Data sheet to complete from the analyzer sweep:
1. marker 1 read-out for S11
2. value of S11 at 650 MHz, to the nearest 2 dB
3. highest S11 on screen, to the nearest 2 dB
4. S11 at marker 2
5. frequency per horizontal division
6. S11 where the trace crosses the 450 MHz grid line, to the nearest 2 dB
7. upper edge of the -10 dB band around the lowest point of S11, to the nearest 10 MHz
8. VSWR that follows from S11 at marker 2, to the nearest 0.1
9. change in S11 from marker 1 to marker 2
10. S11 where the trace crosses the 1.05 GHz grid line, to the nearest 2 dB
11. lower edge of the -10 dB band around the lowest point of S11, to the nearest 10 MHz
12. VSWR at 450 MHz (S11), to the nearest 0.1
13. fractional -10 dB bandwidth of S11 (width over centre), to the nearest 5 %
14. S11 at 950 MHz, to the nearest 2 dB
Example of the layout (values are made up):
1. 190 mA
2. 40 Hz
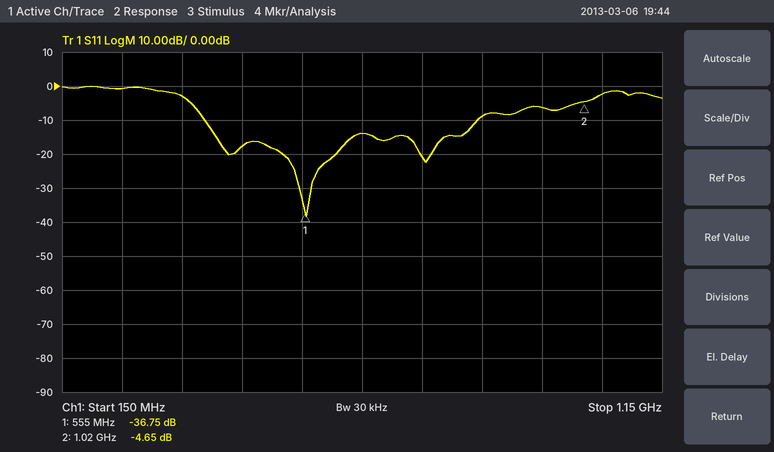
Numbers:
1. -36.75 dB
2. -14 dB
3. 0 dB
4. -4.65 dB
5. 100 MHz
6. -18 dB
7. 840 MHz
8. 3.8
9. 32.10 dB
10. -2 dB
11. 390 MHz
12. 1.3
13. 75 %
14. -6 dB
